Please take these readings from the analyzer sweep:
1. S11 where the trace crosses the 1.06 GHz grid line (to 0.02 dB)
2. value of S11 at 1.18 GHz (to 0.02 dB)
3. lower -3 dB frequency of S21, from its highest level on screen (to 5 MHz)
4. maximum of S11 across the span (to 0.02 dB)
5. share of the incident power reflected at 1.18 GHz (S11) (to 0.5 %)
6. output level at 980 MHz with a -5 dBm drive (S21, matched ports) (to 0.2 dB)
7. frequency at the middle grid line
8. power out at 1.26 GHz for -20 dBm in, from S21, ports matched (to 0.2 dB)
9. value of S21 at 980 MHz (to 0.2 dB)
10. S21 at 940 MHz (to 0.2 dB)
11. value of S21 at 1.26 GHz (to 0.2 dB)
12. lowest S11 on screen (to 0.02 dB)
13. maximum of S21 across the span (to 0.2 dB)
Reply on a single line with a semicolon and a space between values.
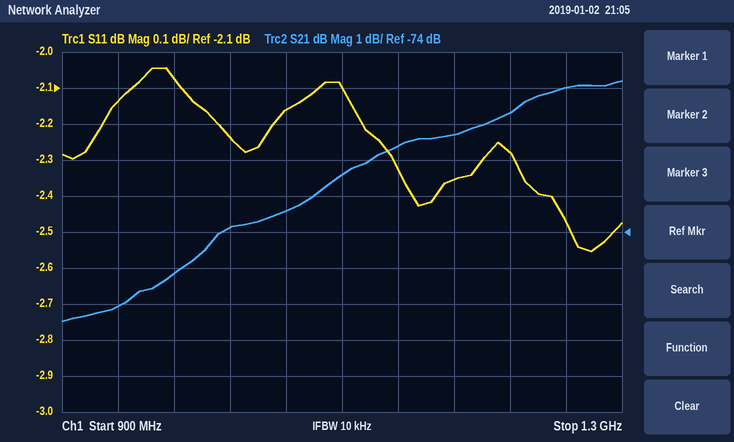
-2.16 dB; -2.36 dB; 1.085 GHz; -2.04 dB; 58.0 %; -80.2 dBm; 1.1 GHz; -90.0 dBm; -75.2 dB; -76.0 dB; -70.0 dB; -2.56 dB; -69.8 dB
